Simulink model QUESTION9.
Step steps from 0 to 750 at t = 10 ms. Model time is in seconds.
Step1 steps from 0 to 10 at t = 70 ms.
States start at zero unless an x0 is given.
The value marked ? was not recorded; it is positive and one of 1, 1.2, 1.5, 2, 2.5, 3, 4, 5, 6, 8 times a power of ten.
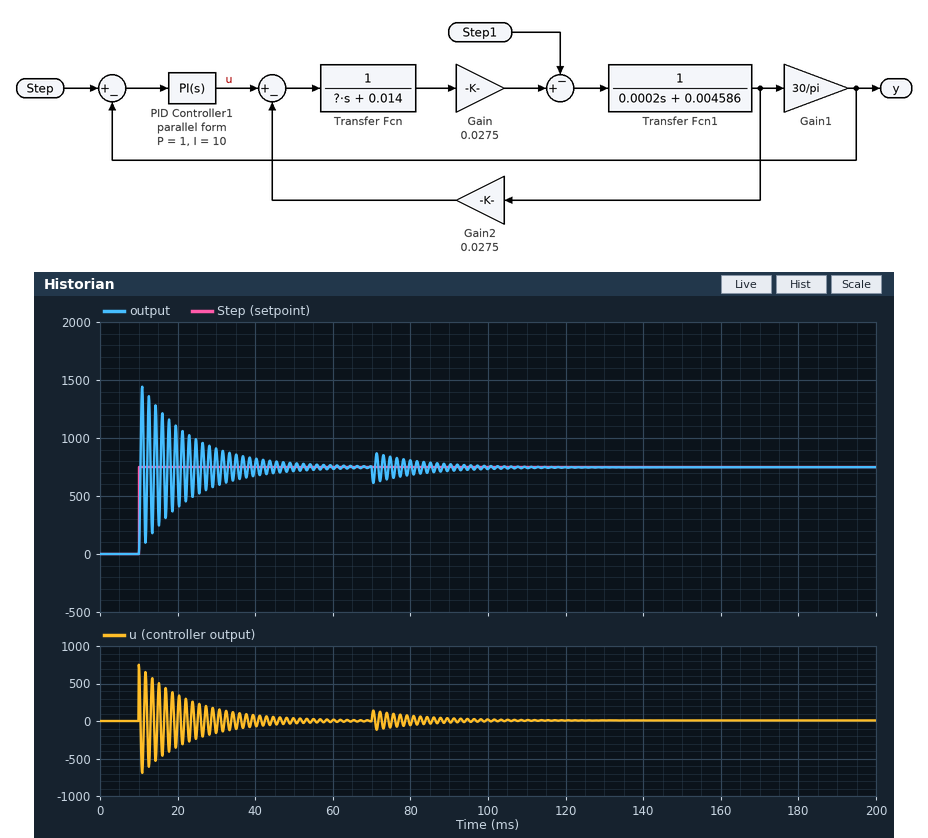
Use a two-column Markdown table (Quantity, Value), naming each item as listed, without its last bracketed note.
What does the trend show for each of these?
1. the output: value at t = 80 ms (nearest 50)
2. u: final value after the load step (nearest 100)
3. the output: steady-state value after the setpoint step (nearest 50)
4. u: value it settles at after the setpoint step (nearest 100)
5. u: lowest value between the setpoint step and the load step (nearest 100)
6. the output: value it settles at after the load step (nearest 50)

| Quantity | Value |
|---|---|
| the output: value at t = 80 ms | 800 |
| u: final value after the load step | 0 |
| the output: steady-state value after the setpoint step | 750 |
| u: value it settles at after the setpoint step | 0 |
| u: lowest value between the setpoint step and the load step | -700 |
| the output: value it settles at after the load step | 750 |
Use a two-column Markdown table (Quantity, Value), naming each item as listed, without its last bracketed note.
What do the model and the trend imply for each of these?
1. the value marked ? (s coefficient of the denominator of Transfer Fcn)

| Quantity | Value |
|---|---|
| the value marked ? | 0.0001 |
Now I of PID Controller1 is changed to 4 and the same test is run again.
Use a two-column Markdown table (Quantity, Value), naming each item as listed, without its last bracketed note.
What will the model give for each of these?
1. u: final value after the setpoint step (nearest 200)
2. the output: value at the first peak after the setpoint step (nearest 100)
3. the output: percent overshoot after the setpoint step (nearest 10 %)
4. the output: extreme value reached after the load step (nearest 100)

| Quantity | Value |
|---|---|
| u: final value after the setpoint step | 0 |
| the output: value at the first peak after the setpoint step | 1400 |
| the output: percent overshoot after the setpoint step | 90 % |
| the output: extreme value reached after the load step | 600 |
